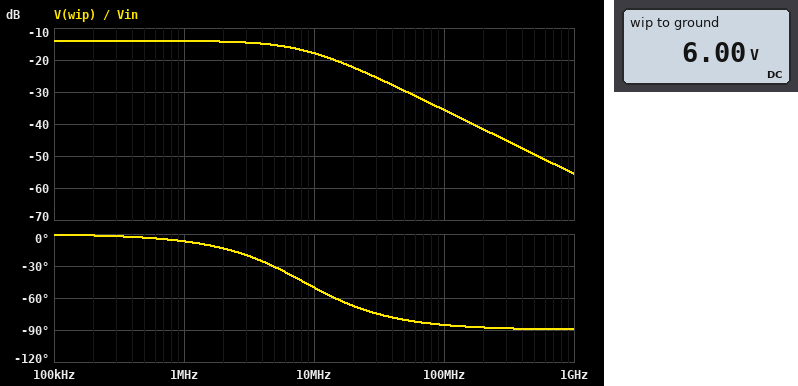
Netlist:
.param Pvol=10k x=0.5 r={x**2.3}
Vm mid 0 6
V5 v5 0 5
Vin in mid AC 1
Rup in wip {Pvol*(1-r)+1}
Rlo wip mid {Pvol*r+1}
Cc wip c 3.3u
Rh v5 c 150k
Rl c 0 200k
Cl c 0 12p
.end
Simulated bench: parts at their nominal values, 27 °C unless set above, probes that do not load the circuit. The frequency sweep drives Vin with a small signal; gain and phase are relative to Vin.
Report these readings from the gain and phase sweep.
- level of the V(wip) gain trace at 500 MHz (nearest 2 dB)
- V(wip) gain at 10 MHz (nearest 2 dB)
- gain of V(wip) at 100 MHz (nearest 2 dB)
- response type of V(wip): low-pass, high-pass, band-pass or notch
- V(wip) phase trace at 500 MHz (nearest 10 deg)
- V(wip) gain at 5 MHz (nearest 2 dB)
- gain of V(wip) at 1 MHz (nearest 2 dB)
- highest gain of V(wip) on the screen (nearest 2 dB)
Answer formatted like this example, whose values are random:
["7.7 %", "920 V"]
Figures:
["-50 dB", "-18 dB", "-36 dB", "low-pass", "-90 deg", "-16 dB", "-14 dB", "-14 dB"]
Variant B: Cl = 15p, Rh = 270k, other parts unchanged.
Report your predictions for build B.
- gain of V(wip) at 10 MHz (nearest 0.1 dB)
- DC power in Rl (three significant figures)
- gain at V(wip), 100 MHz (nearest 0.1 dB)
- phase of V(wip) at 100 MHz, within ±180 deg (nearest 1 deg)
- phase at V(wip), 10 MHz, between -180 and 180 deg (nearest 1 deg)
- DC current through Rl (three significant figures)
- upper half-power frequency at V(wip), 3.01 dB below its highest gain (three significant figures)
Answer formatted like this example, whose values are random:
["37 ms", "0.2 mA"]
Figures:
["-19.1 dB", "22.6 µW", "-37.5 dB", "-86 deg", "-56 deg", "10.6 µA", "6.65 MHz"]
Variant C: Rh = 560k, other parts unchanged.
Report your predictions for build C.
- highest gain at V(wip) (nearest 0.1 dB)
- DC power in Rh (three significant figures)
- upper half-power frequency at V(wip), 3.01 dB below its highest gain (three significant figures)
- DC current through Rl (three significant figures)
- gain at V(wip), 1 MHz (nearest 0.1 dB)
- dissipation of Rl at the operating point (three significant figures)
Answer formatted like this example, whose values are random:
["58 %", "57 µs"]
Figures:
["-13.9 dB", "24.2 µW", "8.28 MHz", "6.58 µA", "-14.0 dB", "8.66 µW"]
